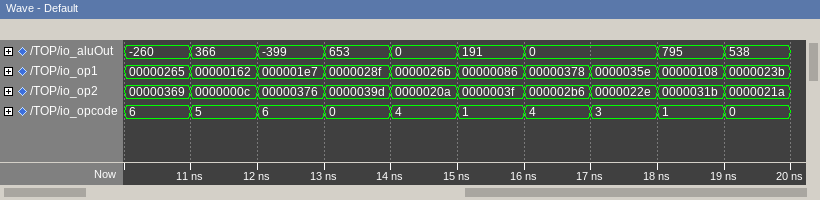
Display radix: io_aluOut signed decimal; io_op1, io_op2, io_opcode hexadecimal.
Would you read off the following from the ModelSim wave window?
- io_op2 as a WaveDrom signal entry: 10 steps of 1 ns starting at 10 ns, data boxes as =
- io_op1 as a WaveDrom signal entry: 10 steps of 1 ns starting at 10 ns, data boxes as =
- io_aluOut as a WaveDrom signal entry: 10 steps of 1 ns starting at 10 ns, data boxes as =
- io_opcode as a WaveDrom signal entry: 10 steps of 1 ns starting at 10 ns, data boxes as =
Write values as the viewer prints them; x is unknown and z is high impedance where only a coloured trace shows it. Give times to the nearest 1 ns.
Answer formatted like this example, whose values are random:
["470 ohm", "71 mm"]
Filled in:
["{name: 'io_op2', wave: '==========', data: '00000369 0000000c 00000376 0000039d 0000020a 0000003f 000002b6 0000022e 0000031b 0000021a'}", "{name: 'io_op1', wave: '==========', data: '00000265 00000162 000001e7 0000028f 0000026b 00000086 00000378 0000035e 00000108 0000023b'}", "{name: 'io_aluOut', wave: '=======.==', data: '-260 366 -399 653 0 191 0 795 538'}", "{name: 'io_opcode', wave: '==========', data: '6 5 6 0 4 1 4 3 1 0'}"]
